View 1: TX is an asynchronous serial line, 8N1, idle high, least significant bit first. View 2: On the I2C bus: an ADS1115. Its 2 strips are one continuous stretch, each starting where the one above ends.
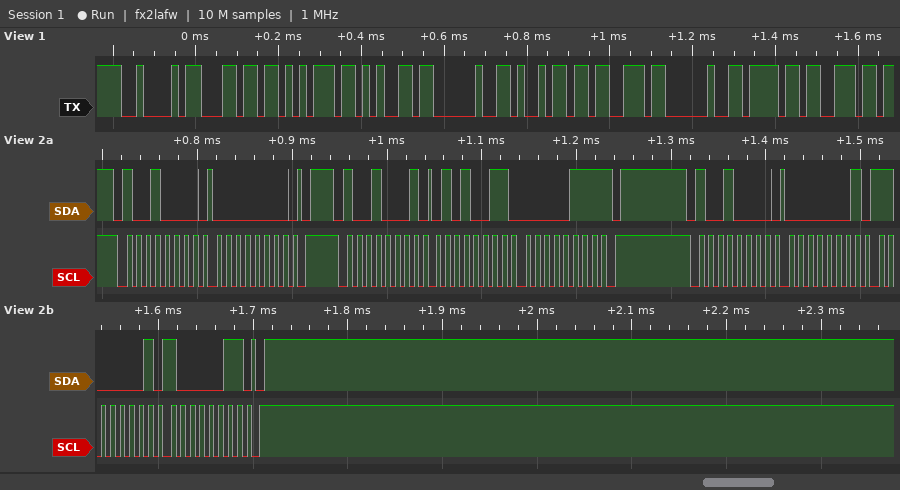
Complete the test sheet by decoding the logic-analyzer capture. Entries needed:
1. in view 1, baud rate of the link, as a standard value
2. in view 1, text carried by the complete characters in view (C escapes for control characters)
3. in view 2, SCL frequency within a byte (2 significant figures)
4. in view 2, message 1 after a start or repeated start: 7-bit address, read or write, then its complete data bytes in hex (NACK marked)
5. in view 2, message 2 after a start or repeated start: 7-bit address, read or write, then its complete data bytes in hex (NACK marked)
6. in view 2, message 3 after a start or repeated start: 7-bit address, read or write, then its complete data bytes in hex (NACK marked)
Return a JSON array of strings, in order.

["57600 baud", "\"Blue is on\"", "100 kHz", "0x48 write: 00", "0x48 read: 53 07 NACK", "0x48 write: 01 C1 83"]
